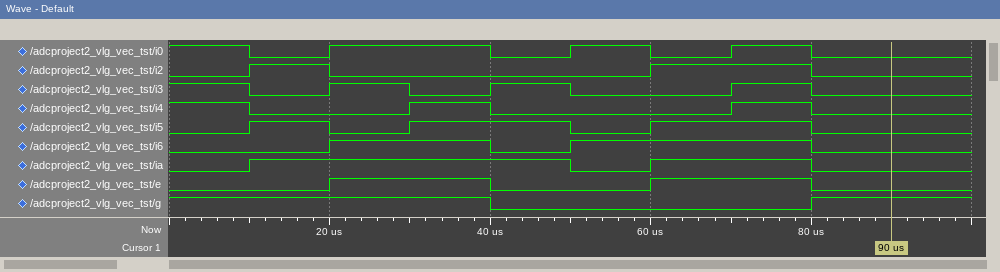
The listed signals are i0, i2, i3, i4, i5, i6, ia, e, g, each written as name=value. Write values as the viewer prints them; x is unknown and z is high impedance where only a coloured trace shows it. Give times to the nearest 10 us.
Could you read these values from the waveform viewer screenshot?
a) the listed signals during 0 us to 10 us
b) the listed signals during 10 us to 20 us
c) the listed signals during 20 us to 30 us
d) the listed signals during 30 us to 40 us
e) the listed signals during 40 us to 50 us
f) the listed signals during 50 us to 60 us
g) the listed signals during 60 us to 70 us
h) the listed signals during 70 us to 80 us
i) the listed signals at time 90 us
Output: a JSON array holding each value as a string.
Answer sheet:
["i0=1, i2=0, i3=1, i4=1, i5=0, i6=0, ia=0, e=0, g=1", "i0=0, i2=1, i3=0, i4=0, i5=1, i6=0, ia=1, e=0, g=1", "i0=1, i2=0, i3=1, i4=0, i5=0, i6=1, ia=1, e=1, g=1", "i0=1, i2=0, i3=0, i4=1, i5=1, i6=1, ia=1, e=1, g=1", "i0=0, i2=0, i3=1, i4=0, i5=1, i6=0, ia=1, e=0, g=0", "i0=1, i2=0, i3=0, i4=0, i5=0, i6=1, ia=0, e=0, g=0", "i0=0, i2=1, i3=0, i4=0, i5=1, i6=1, ia=1, e=1, g=0", "i0=1, i2=1, i3=1, i4=1, i5=1, i6=1, ia=1, e=1, g=0", "i0=0, i2=0, i3=0, i4=0, i5=0, i6=0, ia=0, e=0, g=1"]
